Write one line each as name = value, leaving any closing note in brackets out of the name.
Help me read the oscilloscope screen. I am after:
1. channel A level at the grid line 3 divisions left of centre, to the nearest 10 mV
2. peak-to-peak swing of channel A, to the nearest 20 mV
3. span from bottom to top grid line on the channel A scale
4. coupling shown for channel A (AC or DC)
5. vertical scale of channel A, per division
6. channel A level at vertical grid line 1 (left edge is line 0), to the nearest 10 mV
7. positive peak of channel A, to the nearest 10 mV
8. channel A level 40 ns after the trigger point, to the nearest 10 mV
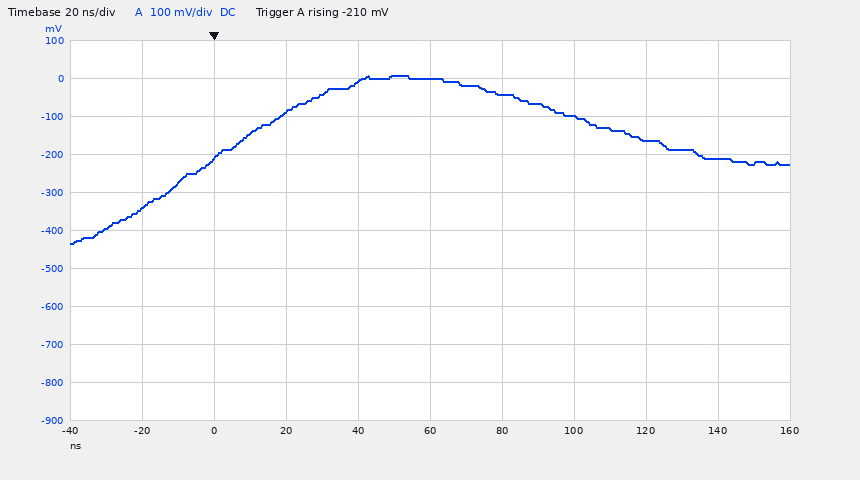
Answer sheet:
channel A level at the grid line 3 divisions left of centre, to the nearest 10 mV = -210 mV
peak-to-peak swing of channel A, to the nearest 20 mV = 440 mV
span from bottom to top grid line on the channel A scale = 1 V
coupling shown for channel A = DC
vertical scale of channel A, per division = 100 mV
channel A level at vertical grid line 1 (left edge is line 0), to the nearest 10 mV = -340 mV
positive peak of channel A, to the nearest 10 mV = 10 mV
channel A level 40 ns after the trigger point, to the nearest 10 mV = -10 mV
